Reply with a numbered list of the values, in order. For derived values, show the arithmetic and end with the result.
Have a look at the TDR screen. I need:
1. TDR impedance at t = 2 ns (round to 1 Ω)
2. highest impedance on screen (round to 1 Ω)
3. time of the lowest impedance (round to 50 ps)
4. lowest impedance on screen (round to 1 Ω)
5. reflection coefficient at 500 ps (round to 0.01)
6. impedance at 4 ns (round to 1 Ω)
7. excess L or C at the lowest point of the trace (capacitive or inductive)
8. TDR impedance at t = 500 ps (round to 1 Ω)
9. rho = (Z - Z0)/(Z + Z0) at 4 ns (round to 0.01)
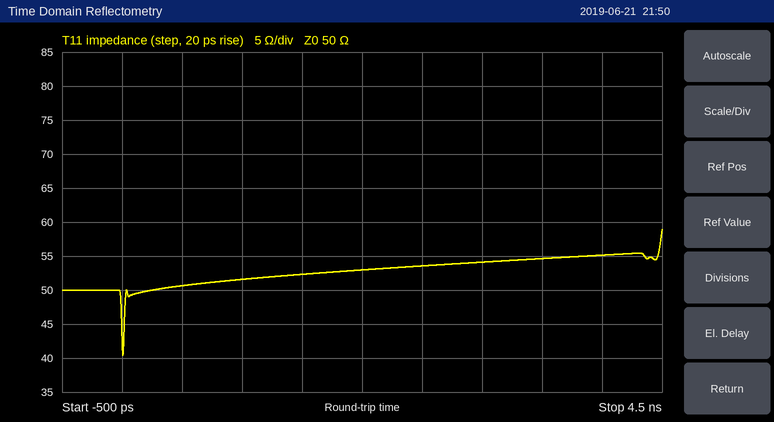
1. 53 Ω
2. 59 Ω
3. 0 ps
4. 40 Ω
5. (51 − 50)/(51 + 50) ≈ +0.01
6. 55 Ω
7. capacitive
8. 51 Ω
9. (55 − 50)/(55 + 50) ≈ +0.05
